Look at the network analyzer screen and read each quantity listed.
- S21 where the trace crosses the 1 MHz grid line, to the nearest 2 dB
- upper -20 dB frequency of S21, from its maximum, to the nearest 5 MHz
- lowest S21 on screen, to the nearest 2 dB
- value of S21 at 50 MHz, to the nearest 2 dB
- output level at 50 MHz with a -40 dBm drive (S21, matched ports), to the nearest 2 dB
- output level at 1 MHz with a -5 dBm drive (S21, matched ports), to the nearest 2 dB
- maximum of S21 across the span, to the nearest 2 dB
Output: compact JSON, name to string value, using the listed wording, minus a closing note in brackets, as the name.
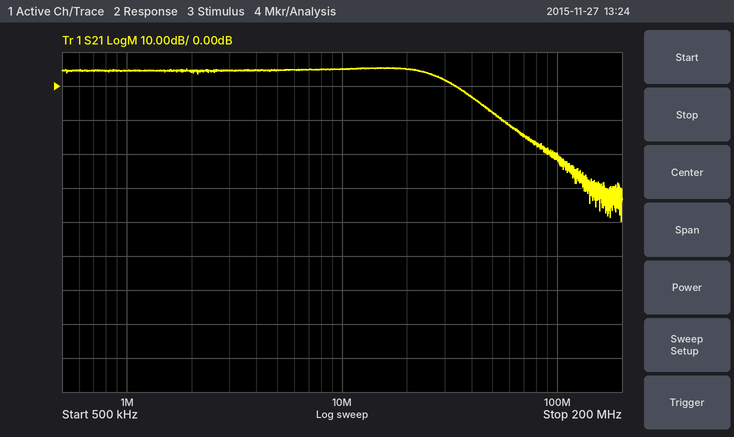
{"S21 where the trace crosses the 1 MHz grid line, to the nearest 2 dB": "4 dB", "upper -20 dB frequency of S21, from its maximum, to the nearest 5 MHz": "70 MHz", "lowest S21 on screen, to the nearest 2 dB": "-40 dB", "value of S21 at 50 MHz, to the nearest 2 dB": "-8 dB", "output level at 50 MHz with a -40 dBm drive (S21, matched ports), to the nearest 2 dB": "-48 dBm", "output level at 1 MHz with a -5 dBm drive (S21, matched ports), to the nearest 2 dB": "0 dBm", "maximum of S21 across the span, to the nearest 2 dB": "6 dB"}
